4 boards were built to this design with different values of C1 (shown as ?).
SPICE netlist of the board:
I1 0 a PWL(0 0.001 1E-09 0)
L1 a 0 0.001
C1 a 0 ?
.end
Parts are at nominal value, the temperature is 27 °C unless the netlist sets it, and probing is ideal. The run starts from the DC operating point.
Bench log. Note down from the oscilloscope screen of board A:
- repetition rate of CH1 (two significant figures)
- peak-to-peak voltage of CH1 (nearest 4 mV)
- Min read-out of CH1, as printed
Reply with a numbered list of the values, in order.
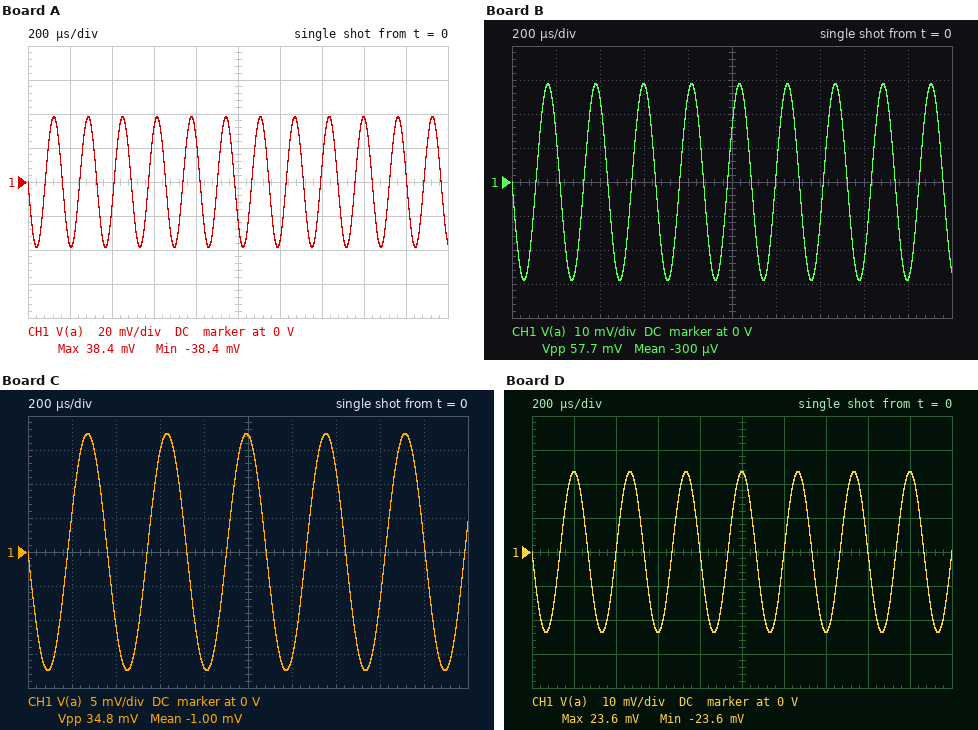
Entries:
1. 6.1 kHz
2. 76 mV
3. -38.4 mV
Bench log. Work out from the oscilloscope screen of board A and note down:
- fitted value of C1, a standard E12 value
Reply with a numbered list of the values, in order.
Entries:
1. 680 nF
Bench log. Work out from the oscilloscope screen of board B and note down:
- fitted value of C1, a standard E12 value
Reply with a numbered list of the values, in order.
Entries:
1. 1.2 µF
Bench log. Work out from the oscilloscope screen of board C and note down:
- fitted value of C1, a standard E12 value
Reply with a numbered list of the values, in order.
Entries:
1. 3.3 µF
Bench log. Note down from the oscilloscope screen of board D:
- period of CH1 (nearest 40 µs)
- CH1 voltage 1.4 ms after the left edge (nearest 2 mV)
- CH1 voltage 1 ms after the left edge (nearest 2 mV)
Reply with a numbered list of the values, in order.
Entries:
1. 280 µs
2. -24 mV
3. 24 mV
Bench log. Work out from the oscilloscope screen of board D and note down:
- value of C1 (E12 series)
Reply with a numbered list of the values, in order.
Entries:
1. 1.8 µF
